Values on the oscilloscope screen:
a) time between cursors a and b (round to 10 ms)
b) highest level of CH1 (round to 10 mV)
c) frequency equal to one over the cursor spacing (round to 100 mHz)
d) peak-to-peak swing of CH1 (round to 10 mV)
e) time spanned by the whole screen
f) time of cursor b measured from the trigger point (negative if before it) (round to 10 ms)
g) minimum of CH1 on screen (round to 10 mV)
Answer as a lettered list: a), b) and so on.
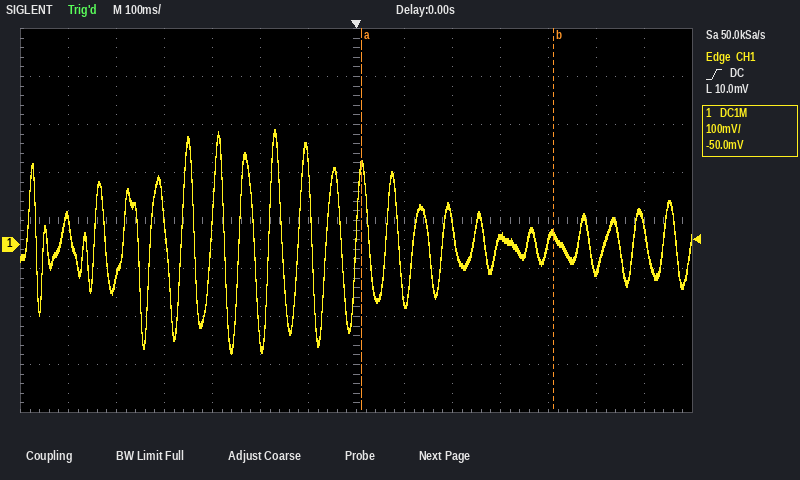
a) 400 ms
b) 240 mV
c) 2.5 Hz
d) 470 mV
e) 1.4 s
f) +410 ms
g) -230 mV
